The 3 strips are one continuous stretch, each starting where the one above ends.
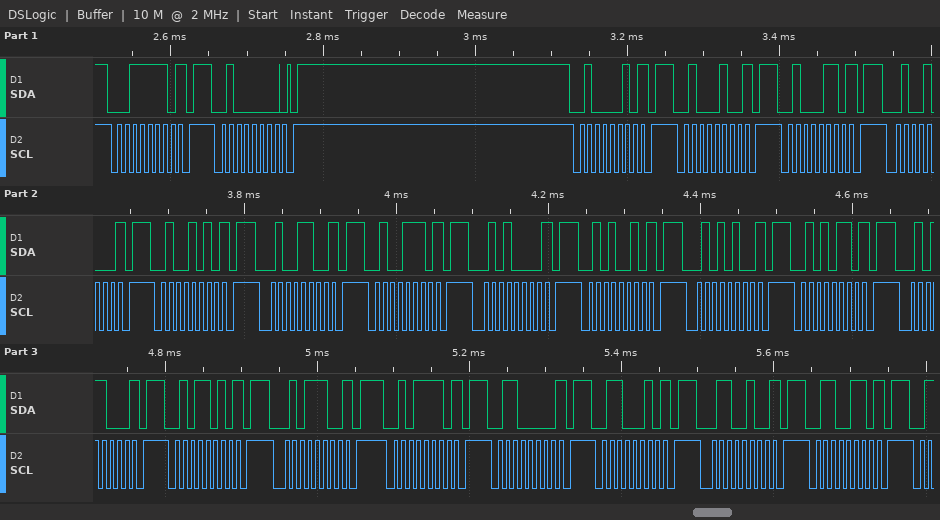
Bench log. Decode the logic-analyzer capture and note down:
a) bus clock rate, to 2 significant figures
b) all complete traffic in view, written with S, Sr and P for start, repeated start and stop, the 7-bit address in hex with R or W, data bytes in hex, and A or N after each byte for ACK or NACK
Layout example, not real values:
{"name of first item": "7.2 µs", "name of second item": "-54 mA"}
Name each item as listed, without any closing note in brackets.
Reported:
{"bus clock rate, to 2 significant figures": "100 kHz", "all complete traffic in view, written with S, Sr and P for start, repeated start and stop, the 7-bit address in hex with R or W, data bytes in hex, and A or N after each byte for ACK or NACK": "S 1FW N P S 20W A P S 21W N P S 22W N P S 23W N P S 24W N P S 25W N P S 26W N P S 27W N P S 28W N P S 29W N P S 2AW N P S 2BW N P S 2CW N P S 2DW N P S 2EW N P S 2FW N P S 30W N P S 31W N P S 32W N P S 33W N P"}
